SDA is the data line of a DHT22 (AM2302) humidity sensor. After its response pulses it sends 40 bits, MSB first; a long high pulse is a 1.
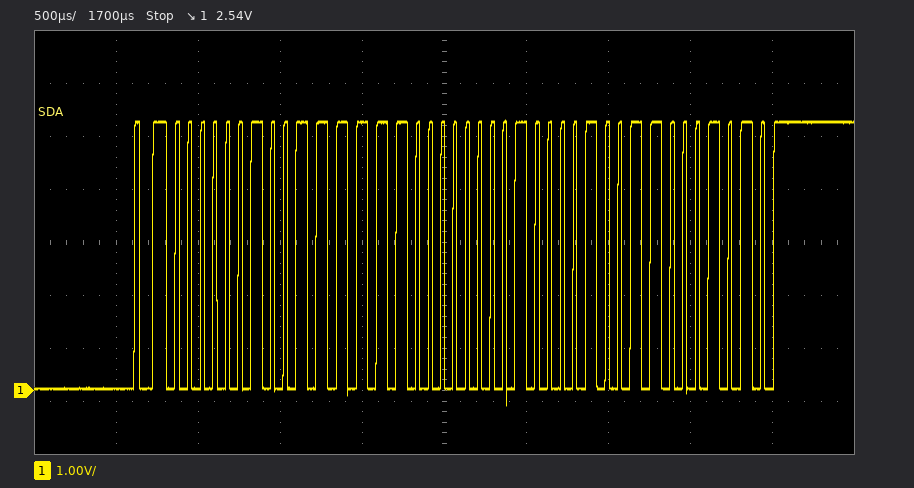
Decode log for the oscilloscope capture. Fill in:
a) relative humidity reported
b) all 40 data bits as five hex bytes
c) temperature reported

63.8 %
02 7E 01 09 8A
26.5 °C
